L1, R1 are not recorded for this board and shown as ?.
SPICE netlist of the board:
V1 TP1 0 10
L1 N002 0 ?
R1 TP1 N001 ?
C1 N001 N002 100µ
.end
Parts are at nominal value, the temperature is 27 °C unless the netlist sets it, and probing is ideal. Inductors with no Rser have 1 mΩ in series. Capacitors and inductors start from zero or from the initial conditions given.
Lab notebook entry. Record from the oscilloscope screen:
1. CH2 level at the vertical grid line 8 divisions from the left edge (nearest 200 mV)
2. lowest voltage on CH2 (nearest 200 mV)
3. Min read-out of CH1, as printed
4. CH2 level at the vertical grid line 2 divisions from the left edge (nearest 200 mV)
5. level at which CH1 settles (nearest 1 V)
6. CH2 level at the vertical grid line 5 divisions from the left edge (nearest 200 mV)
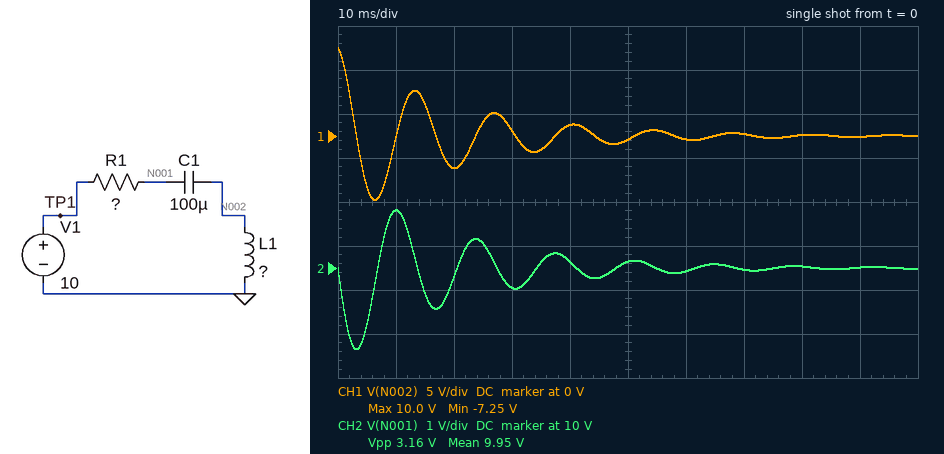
10.0 V
8.2 V
-7.25 V
9.8 V
0 V
10.2 V
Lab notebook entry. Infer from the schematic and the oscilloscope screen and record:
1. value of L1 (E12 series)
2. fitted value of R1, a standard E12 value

47 mH
4.7 Ω
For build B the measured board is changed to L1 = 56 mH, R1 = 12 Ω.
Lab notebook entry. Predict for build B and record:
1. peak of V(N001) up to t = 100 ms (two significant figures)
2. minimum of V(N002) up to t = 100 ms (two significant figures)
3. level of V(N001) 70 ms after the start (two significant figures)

12 V
-5.0 V
10 V
